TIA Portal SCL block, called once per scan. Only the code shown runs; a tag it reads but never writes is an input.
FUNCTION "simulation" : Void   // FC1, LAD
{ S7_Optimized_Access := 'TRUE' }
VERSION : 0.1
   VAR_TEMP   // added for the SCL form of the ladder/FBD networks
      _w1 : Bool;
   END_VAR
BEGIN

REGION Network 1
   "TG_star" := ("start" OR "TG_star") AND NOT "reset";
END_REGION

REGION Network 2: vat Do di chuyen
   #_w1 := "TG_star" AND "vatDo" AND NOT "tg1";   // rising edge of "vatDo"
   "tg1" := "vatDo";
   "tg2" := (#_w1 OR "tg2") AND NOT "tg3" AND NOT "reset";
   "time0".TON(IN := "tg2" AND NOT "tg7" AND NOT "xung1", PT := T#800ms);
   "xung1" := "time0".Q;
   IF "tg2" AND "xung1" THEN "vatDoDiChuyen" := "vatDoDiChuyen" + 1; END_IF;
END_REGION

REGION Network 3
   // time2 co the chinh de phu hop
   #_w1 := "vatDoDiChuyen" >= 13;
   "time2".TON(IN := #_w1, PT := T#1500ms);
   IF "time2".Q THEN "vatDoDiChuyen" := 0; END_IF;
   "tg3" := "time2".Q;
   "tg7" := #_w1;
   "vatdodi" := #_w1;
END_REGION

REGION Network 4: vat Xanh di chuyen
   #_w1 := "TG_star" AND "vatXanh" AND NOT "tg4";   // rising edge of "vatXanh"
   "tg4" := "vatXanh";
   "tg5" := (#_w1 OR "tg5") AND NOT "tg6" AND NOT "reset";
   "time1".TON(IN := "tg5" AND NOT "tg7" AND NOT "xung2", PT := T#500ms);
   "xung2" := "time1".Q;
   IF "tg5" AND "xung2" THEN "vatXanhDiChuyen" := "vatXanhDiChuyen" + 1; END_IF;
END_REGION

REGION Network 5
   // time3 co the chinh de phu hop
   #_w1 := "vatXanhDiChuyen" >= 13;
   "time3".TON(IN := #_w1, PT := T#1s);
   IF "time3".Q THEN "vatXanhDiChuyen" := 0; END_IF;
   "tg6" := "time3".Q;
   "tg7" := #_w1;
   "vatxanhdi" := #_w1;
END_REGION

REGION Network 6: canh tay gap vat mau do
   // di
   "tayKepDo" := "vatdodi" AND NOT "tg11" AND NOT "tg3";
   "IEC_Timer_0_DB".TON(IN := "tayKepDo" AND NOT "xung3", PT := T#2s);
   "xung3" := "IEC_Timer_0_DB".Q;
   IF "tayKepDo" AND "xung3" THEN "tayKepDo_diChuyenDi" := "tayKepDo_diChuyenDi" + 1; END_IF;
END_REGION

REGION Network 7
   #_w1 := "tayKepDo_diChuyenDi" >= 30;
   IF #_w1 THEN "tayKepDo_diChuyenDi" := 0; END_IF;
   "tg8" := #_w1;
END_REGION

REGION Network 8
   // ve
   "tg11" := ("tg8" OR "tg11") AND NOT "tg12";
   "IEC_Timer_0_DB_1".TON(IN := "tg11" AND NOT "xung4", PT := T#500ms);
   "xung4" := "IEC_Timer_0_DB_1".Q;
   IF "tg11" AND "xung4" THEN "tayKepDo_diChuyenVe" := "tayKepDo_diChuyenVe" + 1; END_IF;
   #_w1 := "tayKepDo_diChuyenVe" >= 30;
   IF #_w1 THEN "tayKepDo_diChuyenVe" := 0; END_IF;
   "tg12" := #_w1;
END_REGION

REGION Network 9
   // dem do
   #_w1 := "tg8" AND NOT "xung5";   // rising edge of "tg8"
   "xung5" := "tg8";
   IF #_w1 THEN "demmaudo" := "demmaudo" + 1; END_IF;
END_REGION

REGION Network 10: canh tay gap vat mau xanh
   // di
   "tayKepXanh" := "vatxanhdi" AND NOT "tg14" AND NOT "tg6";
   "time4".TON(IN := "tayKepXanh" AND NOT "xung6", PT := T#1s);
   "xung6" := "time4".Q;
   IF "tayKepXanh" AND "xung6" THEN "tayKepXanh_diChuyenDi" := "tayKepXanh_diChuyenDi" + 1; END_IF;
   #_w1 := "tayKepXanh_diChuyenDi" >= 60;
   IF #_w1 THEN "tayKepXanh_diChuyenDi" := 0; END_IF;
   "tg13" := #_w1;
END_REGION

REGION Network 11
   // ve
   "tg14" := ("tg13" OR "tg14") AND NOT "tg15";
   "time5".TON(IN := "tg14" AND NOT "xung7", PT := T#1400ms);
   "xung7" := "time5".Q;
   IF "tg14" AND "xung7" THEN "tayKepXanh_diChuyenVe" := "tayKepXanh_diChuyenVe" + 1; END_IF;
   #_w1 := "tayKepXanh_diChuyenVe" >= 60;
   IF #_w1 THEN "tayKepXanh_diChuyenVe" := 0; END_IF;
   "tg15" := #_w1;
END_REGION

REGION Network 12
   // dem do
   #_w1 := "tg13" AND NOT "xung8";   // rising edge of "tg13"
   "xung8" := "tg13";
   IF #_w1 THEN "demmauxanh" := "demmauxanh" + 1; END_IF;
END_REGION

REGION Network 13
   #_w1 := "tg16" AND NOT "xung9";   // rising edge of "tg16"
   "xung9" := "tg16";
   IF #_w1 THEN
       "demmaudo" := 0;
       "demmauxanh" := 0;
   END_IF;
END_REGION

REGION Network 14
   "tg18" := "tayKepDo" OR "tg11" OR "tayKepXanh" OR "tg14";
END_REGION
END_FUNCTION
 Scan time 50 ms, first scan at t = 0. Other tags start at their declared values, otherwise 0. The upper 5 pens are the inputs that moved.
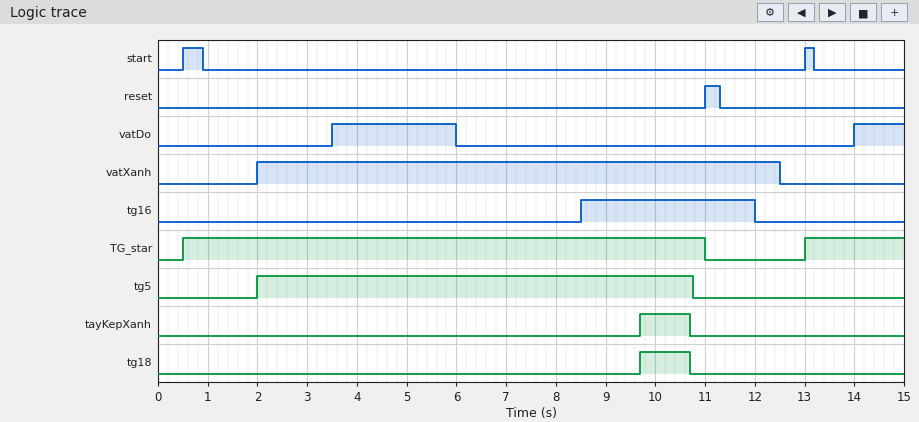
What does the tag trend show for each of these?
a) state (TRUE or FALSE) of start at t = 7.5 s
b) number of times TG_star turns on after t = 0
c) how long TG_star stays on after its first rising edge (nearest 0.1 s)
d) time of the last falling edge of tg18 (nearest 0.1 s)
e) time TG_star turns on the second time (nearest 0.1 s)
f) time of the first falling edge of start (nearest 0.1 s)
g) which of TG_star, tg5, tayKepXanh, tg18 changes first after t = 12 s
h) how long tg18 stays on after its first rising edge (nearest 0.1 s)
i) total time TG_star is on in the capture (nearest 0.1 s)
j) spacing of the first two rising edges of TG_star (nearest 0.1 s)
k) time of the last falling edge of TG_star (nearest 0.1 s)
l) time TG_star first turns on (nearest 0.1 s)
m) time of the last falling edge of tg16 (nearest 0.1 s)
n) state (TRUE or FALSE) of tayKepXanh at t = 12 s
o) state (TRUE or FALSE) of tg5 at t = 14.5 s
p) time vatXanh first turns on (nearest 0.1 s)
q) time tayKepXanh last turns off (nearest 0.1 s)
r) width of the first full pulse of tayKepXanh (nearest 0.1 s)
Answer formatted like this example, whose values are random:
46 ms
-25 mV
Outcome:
FALSE
2
10.5 s
10.7 s
13.0 s
0.9 s
TG_star
1.0 s
12.5 s
12.5 s
11.0 s
0.5 s
12.0 s
FALSE
FALSE
2.0 s
10.7 s
1.0 s
